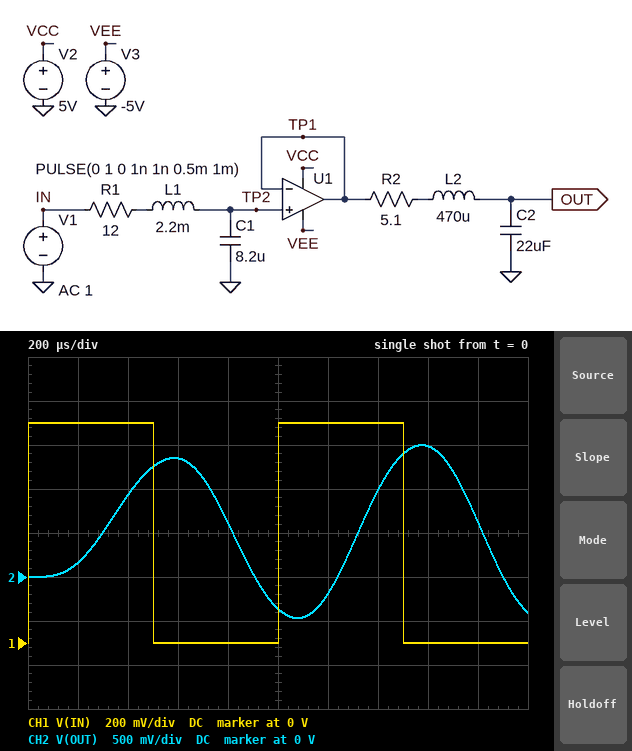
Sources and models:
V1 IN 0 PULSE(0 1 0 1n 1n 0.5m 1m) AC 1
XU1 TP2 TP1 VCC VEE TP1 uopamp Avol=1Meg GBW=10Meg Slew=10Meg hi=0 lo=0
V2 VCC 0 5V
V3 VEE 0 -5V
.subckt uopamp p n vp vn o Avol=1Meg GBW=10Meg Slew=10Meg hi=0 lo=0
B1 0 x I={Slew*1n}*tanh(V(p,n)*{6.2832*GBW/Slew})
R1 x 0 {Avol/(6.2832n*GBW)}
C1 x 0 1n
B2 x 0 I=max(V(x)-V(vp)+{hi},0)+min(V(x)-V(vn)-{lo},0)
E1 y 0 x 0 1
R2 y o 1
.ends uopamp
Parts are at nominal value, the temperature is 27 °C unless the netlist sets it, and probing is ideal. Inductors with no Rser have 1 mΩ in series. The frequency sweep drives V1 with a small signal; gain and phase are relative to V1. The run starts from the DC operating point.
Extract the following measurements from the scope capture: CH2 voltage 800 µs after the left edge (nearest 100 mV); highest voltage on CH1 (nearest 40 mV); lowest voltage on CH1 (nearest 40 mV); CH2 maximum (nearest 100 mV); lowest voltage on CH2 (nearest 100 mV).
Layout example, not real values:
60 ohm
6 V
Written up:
600 mV
1.00 V
0 V
1.5 V
-500 mV
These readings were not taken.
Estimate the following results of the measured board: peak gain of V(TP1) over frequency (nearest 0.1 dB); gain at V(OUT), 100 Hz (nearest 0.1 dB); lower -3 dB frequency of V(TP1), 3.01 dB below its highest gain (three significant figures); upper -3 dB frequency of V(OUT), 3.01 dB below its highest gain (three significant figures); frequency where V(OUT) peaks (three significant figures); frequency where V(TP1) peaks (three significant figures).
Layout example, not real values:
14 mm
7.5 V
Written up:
3.3 dB
0.1 dB
265 Hz
1.36 kHz
1.01 kHz
1.01 kHz
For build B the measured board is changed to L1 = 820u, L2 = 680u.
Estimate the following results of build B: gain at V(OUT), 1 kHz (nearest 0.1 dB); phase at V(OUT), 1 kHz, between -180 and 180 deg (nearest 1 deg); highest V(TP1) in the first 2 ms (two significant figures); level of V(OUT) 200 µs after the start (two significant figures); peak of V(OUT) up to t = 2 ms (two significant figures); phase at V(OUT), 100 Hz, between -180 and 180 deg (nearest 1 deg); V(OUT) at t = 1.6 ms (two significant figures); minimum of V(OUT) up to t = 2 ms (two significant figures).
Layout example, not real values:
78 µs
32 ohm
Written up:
2.1 dB
-100 deg
1.1 V
230 mV
1.3 V
-8 deg
1.2 V
-290 mV
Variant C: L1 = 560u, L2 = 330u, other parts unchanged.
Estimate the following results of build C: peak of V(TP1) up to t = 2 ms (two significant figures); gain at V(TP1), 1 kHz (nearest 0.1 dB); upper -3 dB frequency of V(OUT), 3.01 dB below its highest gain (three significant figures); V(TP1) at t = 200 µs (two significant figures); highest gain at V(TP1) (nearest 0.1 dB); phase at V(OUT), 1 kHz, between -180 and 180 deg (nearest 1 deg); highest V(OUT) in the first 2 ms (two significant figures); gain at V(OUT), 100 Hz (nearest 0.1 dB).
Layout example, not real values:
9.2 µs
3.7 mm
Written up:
1.0 V
-0.2 dB
1.71 kHz
940 mV
0 dB
-82 deg
1.1 V
0 dB
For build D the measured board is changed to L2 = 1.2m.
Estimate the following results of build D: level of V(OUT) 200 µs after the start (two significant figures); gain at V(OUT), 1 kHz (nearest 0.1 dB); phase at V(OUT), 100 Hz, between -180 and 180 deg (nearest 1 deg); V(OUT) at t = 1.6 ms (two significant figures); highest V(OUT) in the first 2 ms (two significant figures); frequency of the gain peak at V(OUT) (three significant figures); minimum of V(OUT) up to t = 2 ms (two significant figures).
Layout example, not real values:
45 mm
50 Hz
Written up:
86 mV
6.3 dB
-8 deg
1.6 V
1.8 V
904 Hz
-710 mV
